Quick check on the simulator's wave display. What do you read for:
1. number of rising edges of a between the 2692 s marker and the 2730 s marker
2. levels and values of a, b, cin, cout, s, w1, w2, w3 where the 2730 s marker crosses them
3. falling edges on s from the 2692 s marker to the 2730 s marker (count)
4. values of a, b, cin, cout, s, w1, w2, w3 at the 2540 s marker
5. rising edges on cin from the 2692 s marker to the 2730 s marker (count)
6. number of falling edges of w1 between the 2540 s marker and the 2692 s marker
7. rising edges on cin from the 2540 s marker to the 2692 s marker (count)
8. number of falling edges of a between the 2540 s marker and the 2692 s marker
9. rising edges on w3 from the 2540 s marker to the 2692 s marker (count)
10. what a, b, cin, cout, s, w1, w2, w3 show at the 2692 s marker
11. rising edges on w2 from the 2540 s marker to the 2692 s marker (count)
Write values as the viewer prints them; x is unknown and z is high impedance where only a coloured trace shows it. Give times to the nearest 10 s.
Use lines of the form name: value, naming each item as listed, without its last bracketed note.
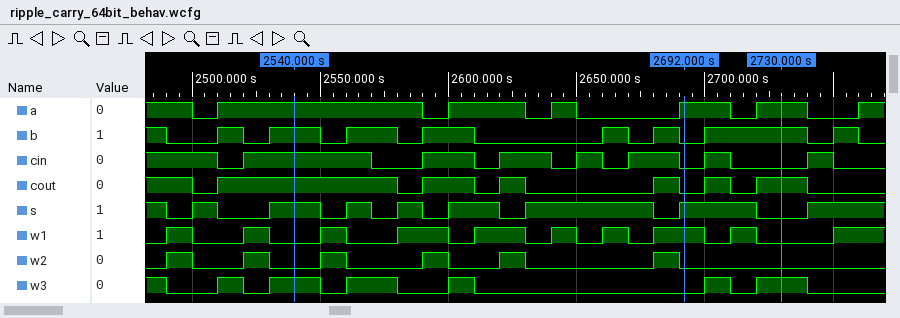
number of rising edges of a between the 2692 s marker and the 2730 s marker: 1
levels and values of a, b, cin, cout, s, w1, w2, w3 where the 2730 s marker crosses them: a=1, b=1, cin=0, cout=1, s=0, w1=0, w2=0, w3=1
falling edges on s from the 2692 s marker to the 2730 s marker: 1
values of a, b, cin, cout, s, w1, w2, w3 at the 2540 s marker: a=1, b=1, cin=1, cout=1, s=1, w1=0, w2=0, w3=1
rising edges on cin from the 2692 s marker to the 2730 s marker: 1
number of falling edges of w1 between the 2540 s marker and the 2692 s marker: 5
rising edges on cin from the 2540 s marker to the 2692 s marker: 4
number of falling edges of a between the 2540 s marker and the 2692 s marker: 3
rising edges on w3 from the 2540 s marker to the 2692 s marker: 2
what a, b, cin, cout, s, w1, w2, w3 show at the 2692 s marker: a=1, b=0, cin=0, cout=0, s=1, w1=1, w2=0, w3=0
rising edges on w2 from the 2540 s marker to the 2692 s marker: 4
